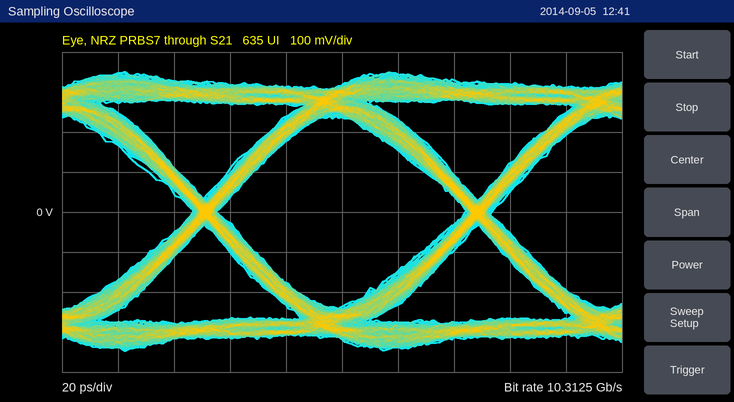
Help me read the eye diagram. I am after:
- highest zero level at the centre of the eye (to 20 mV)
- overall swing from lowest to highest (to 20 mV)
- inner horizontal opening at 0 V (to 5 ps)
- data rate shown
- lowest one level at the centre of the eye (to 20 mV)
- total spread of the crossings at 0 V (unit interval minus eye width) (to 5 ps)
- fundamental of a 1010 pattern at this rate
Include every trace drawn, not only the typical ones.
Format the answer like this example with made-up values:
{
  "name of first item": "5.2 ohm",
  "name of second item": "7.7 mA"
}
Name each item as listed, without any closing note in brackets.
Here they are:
{
  "highest zero level at the centre of the eye": "-240 mV",
  "overall swing from lowest to highest": "700 mV",
  "inner horizontal opening at 0 V": "90 ps",
  "data rate shown": "10.3125 Gb/s",
  "lowest one level at the centre of the eye": "240 mV",
  "total spread of the crossings at 0 V (unit interval minus eye width)": "10 ps",
  "fundamental of a 1010 pattern at this rate": "5.15625 GHz"
}
